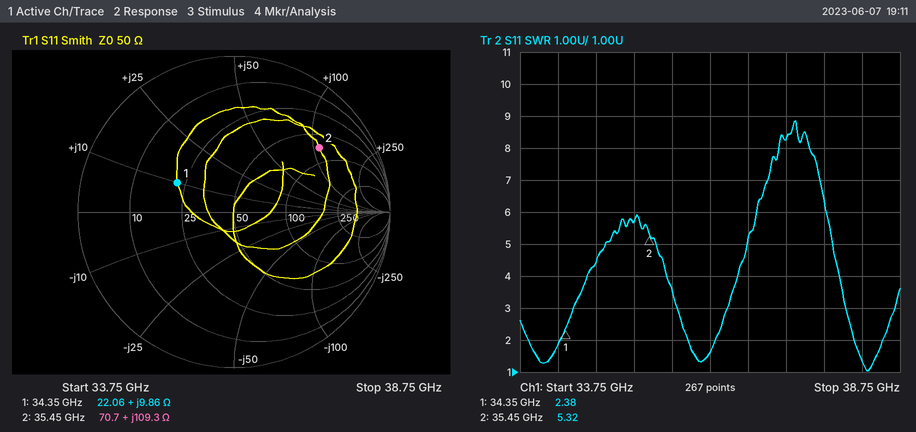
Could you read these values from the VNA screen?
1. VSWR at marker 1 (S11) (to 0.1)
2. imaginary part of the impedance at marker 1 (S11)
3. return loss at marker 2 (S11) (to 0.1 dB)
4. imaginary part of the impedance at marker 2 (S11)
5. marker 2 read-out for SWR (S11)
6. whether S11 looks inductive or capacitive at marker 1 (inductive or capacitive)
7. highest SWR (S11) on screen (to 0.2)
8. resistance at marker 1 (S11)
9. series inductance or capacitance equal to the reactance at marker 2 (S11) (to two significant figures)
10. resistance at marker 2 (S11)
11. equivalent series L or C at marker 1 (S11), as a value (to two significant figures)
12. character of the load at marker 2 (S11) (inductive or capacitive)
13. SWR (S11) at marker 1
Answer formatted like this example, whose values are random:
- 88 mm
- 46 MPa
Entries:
- 2.4
- +9.86 Ω
- 3.3 dB
- +109.3 Ω
- 5.32
- inductive
- 8.8
- 22.06 Ω
- 490 pH
- 70.7 Ω
- 46 pH
- inductive
- 2.38
